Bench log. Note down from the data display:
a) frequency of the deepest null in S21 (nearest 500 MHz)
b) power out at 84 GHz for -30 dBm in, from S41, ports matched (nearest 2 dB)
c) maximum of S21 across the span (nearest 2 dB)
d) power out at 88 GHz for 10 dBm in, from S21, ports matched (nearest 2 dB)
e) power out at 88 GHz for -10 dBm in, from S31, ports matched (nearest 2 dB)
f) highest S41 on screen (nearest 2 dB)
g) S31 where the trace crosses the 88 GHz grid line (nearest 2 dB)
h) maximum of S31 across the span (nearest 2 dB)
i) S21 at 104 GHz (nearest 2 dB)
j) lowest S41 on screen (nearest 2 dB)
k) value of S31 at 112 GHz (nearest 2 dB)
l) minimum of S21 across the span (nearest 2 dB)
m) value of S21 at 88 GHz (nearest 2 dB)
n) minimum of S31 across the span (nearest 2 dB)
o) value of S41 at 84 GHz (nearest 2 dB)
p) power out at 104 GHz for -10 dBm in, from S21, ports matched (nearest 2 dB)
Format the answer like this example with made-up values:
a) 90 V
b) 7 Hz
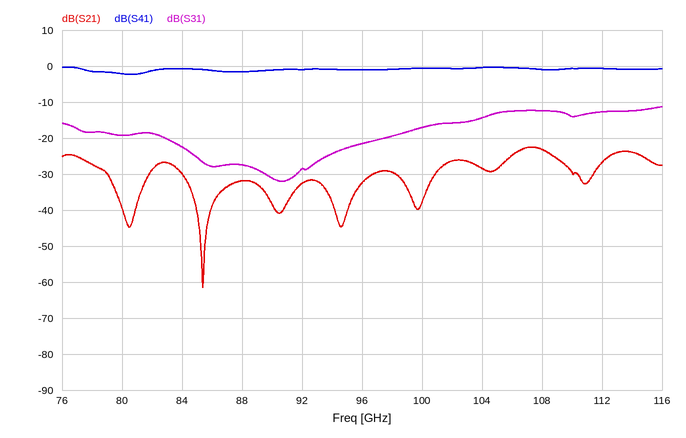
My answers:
a) 85.5 GHz
b) -30 dBm
c) -22 dB
d) -22 dBm
e) -38 dBm
f) 0 dB
g) -28 dB
h) -12 dB
i) -28 dB
j) -2 dB
k) -12 dB
l) -62 dB
m) -32 dB
n) -32 dB
o) 0 dB
p) -38 dBm
